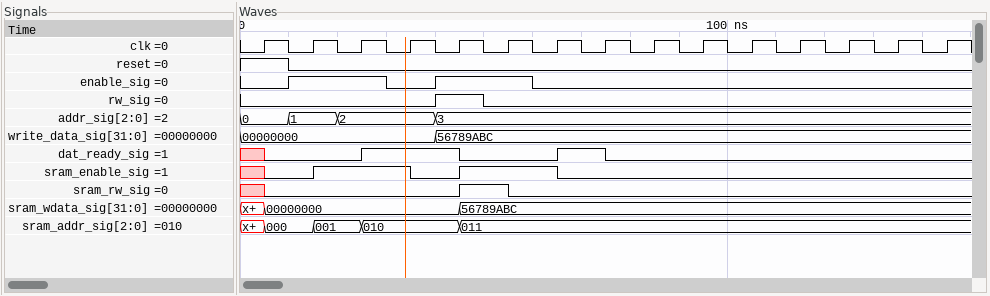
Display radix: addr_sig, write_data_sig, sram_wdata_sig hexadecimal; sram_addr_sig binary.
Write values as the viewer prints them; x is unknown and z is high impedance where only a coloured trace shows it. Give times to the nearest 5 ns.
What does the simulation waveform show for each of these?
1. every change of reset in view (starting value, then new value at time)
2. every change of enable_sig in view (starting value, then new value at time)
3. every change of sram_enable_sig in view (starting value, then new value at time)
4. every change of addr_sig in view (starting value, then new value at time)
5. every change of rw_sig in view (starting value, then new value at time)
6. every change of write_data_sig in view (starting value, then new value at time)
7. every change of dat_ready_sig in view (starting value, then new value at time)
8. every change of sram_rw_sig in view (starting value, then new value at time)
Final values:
1, 0 at 10 ns
0, 1 at 10 ns, 0 at 30 ns, 1 at 40 ns, 0 at 60 ns
x, 0 at 5 ns, 1 at 15 ns, 0 at 35 ns, 1 at 45 ns, 0 at 65 ns
0, 1 at 10 ns, 2 at 20 ns, 3 at 40 ns
0, 1 at 40 ns, 0 at 50 ns
00000000, 56789ABC at 40 ns
x, 0 at 5 ns, 1 at 25 ns, 0 at 45 ns, 1 at 65 ns, 0 at 75 ns
x, 0 at 5 ns, 1 at 45 ns, 0 at 55 ns
